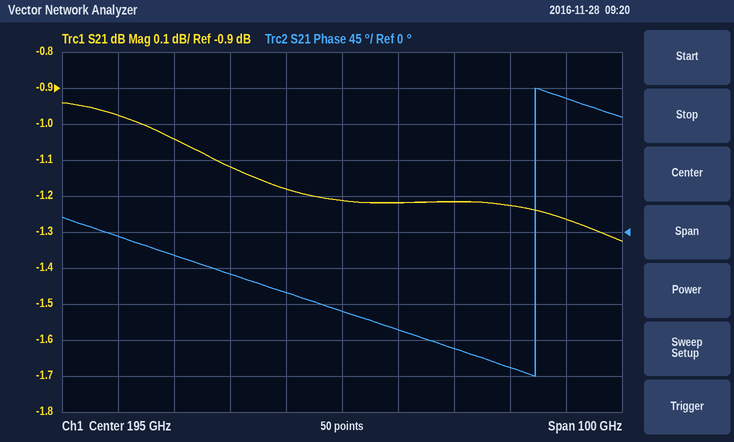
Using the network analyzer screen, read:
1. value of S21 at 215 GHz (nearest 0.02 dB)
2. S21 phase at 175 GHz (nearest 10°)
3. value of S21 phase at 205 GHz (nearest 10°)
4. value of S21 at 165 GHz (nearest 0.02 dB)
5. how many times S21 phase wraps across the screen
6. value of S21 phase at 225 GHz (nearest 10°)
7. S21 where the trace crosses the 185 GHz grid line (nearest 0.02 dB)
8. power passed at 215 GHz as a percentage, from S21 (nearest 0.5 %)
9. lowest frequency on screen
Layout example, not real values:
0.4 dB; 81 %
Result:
-1.22 dB; -50°; -120°; -1.04 dB; 1; -170°; -1.18 dB; 75.5 %; 145 GHz
